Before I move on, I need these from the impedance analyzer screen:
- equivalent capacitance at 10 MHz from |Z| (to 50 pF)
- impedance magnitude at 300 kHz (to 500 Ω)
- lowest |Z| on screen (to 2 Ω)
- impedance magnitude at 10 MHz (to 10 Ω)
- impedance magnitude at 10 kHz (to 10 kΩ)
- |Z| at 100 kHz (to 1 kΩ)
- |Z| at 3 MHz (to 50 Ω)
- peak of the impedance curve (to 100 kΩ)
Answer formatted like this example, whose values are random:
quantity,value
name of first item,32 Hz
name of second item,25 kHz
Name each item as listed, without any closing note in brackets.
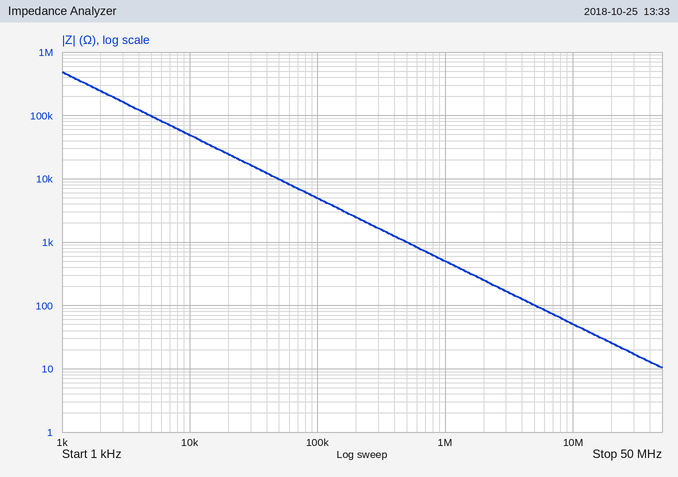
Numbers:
quantity,value
equivalent capacitance at 10 MHz from |Z|,300 pF
impedance magnitude at 300 kHz,1.5 kΩ
lowest |Z| on screen,10 Ω
impedance magnitude at 10 MHz,50 Ω
impedance magnitude at 10 kHz,50 kΩ
|Z| at 100 kHz,5 kΩ
|Z| at 3 MHz,150 Ω
peak of the impedance curve,500 kΩ
